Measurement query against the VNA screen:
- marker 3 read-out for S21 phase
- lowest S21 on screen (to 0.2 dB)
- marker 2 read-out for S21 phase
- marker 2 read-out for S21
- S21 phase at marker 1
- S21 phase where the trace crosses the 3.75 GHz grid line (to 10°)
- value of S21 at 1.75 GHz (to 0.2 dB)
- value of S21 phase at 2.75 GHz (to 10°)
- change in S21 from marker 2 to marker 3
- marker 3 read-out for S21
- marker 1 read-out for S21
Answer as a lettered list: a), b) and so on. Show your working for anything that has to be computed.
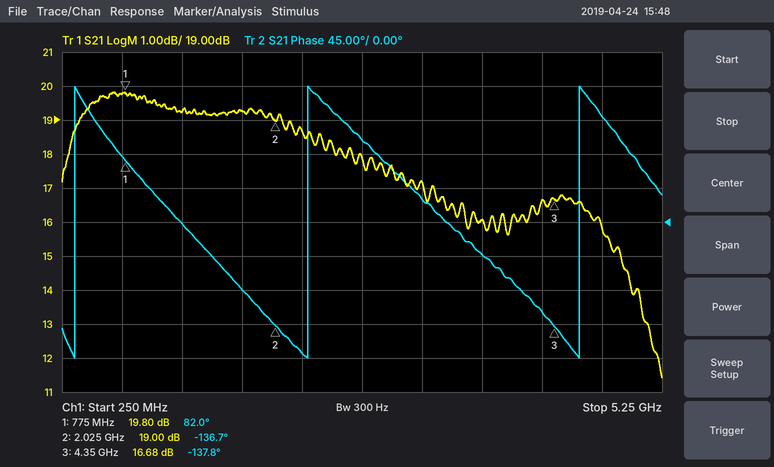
a) -137.8°
b) 11.4 dB
c) -136.7°
d) 19.00 dB
e) 82.0°
f) -40°
g) 19.2 dB
h) 110°
i) 16.68 − (19) = -2.32 dB
j) 16.68 dB
k) 19.80 dB
